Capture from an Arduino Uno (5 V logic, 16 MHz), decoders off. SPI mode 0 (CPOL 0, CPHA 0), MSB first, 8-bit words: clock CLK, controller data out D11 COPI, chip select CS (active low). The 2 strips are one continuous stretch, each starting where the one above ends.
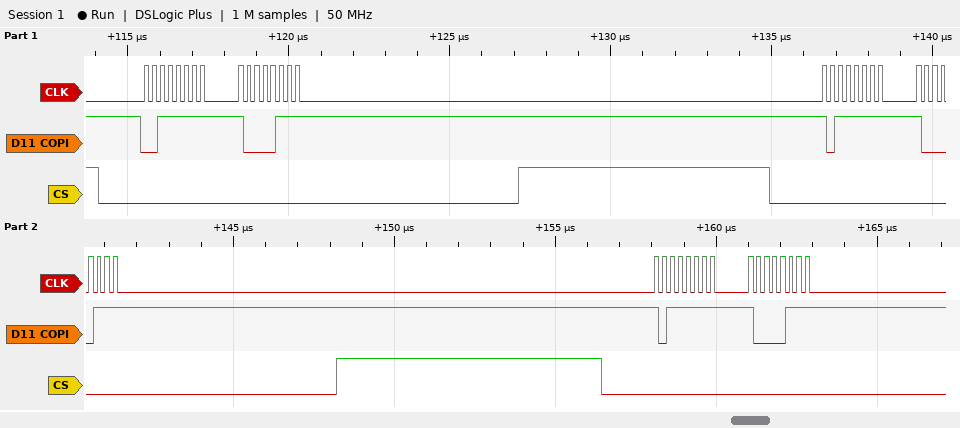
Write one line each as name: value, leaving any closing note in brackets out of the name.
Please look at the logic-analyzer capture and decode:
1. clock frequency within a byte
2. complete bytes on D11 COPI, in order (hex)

clock frequency within a byte: 4 MHz
complete bytes on D11 COPI, in order: 0x3F 0x87 0xBF 0x87 0xBF 0x87
